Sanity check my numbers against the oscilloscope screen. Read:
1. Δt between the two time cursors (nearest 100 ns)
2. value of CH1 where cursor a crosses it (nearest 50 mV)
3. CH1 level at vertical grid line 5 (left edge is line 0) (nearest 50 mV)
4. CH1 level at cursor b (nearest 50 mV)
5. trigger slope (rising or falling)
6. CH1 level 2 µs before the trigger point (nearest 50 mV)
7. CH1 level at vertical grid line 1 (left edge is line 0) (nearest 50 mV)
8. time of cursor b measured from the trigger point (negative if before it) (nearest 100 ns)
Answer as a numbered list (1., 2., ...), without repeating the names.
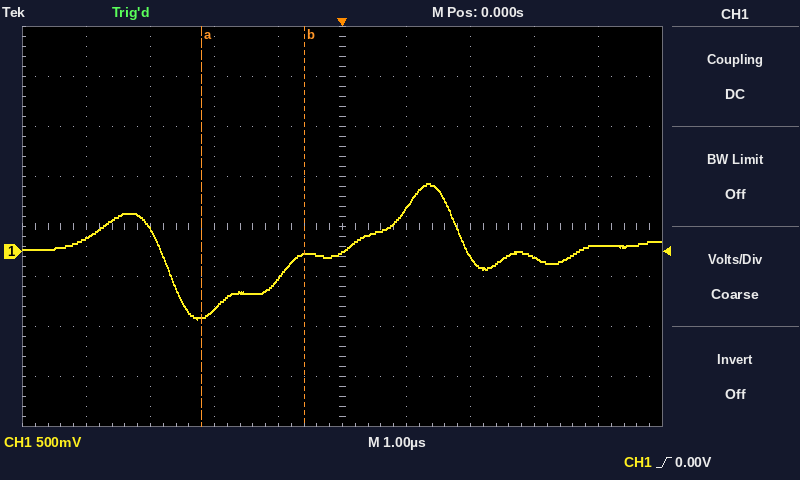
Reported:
1. 1.6 µs
2. -650 mV
3. 0 mV
4. -50 mV
5. rising
6. -600 mV
7. 150 mV
8. -600 ns
